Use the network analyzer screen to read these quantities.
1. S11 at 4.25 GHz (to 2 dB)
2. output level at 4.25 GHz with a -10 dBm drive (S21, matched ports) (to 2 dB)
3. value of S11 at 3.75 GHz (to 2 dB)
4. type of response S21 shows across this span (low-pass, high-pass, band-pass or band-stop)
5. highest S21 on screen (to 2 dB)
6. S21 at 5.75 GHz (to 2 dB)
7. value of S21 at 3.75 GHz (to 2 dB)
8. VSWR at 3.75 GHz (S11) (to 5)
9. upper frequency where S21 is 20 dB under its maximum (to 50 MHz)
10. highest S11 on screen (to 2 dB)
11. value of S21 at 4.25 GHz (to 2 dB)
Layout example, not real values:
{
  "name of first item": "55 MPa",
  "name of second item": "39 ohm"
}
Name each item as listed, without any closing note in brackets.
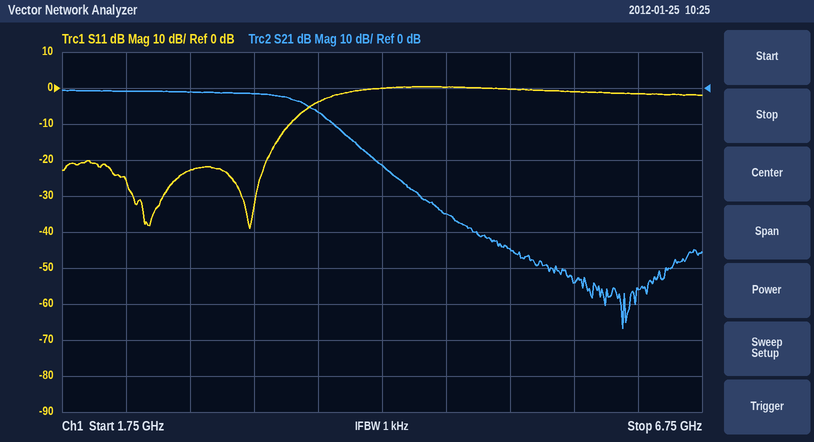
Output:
{
  "S11 at 4.25 GHz": "0 dB",
  "output level at 4.25 GHz with a -10 dBm drive (S21, matched ports)": "-32 dBm",
  "value of S11 at 3.75 GHz": "-4 dB",
  "type of response S21 shows across this span": "low-pass",
  "highest S21 on screen": "0 dB",
  "S21 at 5.75 GHz": "-54 dB",
  "value of S21 at 3.75 GHz": "-6 dB",
  "VSWR at 3.75 GHz (S11)": "5",
  "upper frequency where S21 is 20 dB under its maximum": "4.20 GHz",
  "highest S11 on screen": "0 dB",
  "value of S21 at 4.25 GHz": "-22 dB"
}
